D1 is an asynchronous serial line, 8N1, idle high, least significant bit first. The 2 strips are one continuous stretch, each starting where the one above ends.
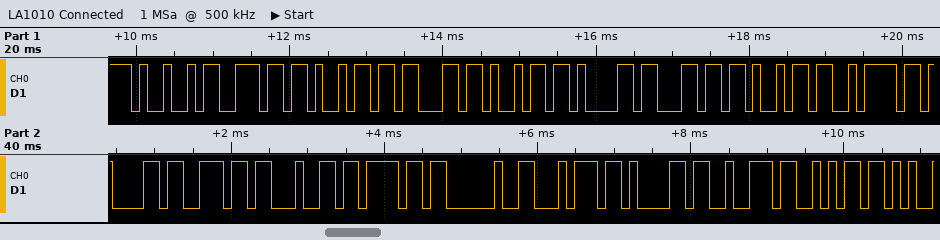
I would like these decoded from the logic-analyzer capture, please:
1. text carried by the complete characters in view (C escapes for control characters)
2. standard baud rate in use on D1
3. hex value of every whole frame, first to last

"Inicializando tarj"
9600 baud
0x49 0x6E 0x69 0x63 0x69 0x61 0x6C 0x69 0x7A 0x61 0x6E 0x64 0x6F 0x20 0x74 0x61 0x72 0x6A
